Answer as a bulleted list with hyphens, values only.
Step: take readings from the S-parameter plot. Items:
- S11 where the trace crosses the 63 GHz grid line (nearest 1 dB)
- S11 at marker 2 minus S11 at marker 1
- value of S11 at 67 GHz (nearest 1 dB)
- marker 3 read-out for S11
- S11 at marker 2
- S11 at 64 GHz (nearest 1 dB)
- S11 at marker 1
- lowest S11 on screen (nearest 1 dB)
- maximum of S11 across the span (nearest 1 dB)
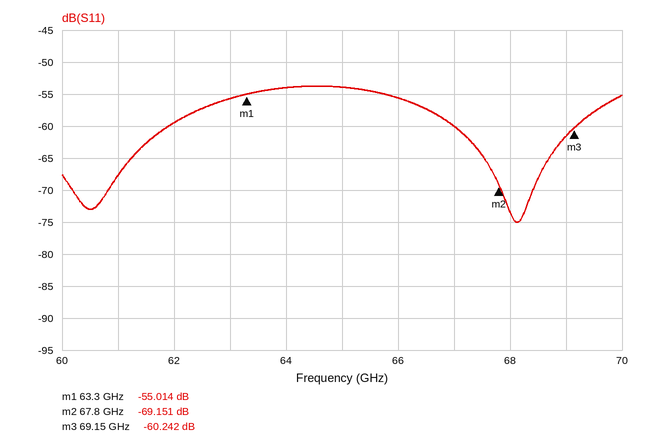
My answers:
- -56 dB
- -14.137 dB
- -60 dB
- -60.242 dB
- -69.151 dB
- -54 dB
- -55.014 dB
- -75 dB
- -54 dB
